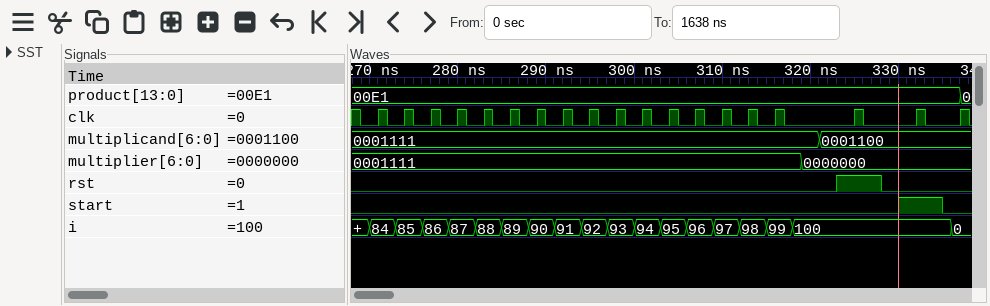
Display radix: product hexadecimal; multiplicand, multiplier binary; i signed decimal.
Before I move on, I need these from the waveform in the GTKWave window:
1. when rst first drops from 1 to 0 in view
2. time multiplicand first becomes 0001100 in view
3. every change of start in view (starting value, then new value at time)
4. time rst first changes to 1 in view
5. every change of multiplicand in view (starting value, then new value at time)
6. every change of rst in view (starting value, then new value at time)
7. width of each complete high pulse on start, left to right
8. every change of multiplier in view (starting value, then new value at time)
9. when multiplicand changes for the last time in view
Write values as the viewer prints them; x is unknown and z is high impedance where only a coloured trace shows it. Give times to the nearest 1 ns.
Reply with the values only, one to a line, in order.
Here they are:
328 ns
321 ns
0, 1 at 330 ns, 0 at 335 ns
323 ns
0001111, 0001100 at 321 ns
0, 1 at 323 ns, 0 at 328 ns
5 ns
0001111, 0000000 at 319 ns
321 ns
